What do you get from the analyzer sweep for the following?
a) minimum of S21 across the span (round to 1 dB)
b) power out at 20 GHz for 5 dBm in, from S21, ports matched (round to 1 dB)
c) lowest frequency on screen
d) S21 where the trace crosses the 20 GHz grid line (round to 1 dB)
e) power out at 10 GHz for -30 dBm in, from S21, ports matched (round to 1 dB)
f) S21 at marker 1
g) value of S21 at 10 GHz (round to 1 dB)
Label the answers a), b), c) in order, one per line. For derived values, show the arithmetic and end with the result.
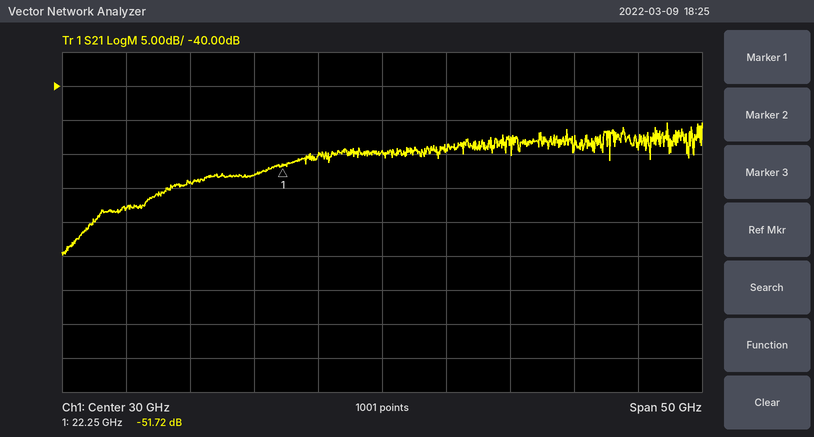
a) -65 dB
b) 5 dBm + (-53 dB) = -48 dBm
c) 5 GHz
d) -53 dB
e) -30 dBm + (-58 dB) = -88 dBm
f) -51.72 dB
g) -58 dB
